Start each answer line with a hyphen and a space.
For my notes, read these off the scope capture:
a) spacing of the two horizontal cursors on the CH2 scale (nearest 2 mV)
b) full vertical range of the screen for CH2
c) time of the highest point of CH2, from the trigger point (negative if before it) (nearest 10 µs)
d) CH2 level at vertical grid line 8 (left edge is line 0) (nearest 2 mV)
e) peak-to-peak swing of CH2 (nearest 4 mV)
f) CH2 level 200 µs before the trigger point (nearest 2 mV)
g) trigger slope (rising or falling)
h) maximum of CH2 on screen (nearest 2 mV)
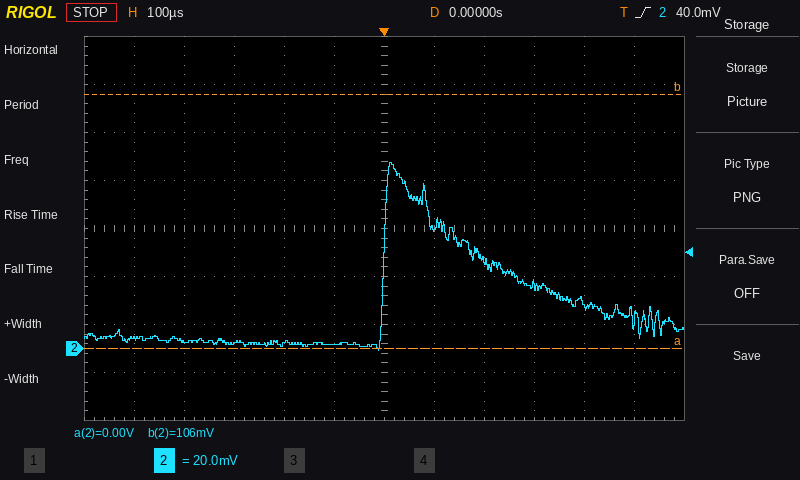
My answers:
- 106 mV
- 160 mV
- +10 µs
- 36 mV
- 80 mV
- 2 mV
- rising
- 78 mV
